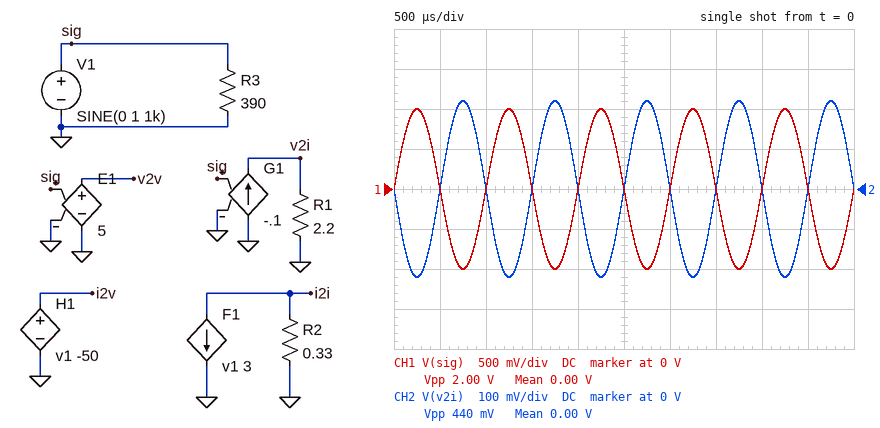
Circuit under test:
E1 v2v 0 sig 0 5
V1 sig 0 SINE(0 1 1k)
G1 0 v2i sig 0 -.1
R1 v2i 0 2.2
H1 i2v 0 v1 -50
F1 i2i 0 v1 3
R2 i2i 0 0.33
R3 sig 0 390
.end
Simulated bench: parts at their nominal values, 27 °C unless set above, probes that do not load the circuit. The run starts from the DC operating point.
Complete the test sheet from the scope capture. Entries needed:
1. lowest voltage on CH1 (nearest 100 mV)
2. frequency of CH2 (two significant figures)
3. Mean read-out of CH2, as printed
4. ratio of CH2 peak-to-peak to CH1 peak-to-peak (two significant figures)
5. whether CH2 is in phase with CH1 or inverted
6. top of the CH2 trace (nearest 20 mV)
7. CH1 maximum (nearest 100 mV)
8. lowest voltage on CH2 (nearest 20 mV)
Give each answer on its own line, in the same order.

-1.0 V
1.0 kHz
0.00 V
0.22
inverted
220 mV
1.0 V
-220 mV
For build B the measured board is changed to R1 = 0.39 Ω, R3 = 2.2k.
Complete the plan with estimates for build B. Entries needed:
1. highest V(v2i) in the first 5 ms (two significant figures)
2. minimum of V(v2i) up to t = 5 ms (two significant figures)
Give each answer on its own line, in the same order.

39 mV
-39 mV
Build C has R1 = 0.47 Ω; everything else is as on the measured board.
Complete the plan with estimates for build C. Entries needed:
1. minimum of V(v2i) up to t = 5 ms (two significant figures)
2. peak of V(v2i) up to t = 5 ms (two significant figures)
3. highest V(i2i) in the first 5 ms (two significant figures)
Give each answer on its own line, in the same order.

-47 mV
47 mV
2.5 mV
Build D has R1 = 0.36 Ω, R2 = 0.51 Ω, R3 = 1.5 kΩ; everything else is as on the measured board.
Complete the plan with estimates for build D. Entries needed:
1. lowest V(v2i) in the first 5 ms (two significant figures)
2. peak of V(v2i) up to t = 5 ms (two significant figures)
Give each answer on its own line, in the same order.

-36 mV
36 mV
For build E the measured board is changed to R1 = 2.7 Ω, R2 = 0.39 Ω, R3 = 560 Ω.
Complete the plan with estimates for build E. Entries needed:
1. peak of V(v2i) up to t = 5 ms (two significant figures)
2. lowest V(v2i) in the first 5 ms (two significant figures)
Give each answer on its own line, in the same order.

270 mV
-270 mV
